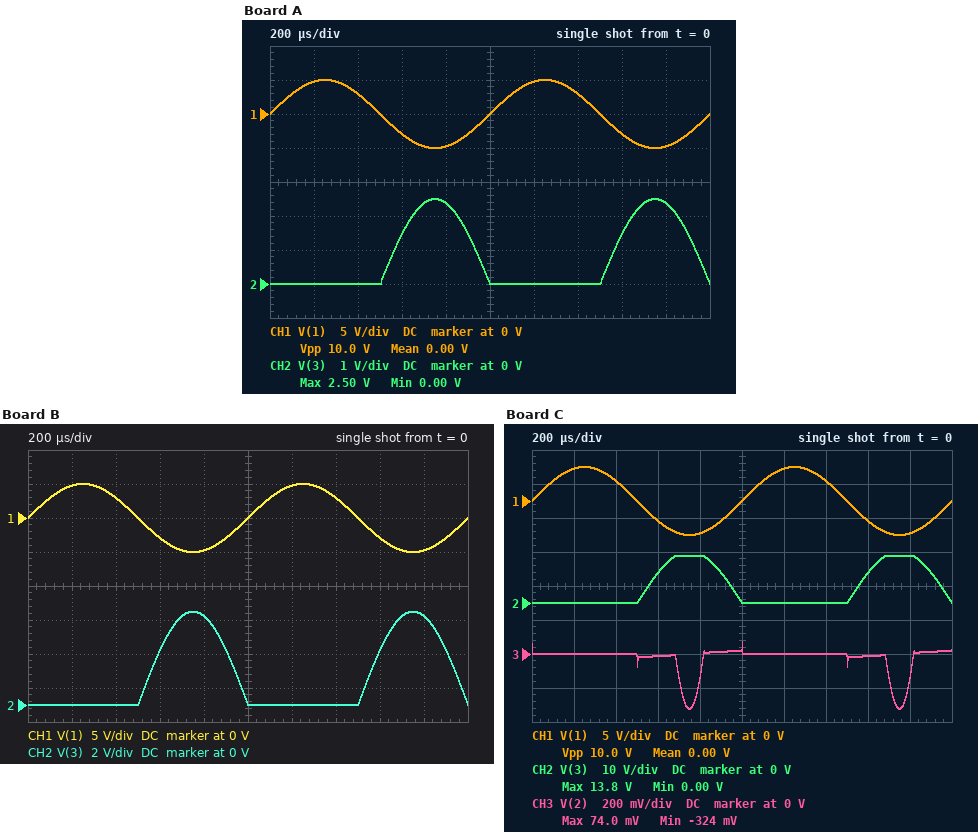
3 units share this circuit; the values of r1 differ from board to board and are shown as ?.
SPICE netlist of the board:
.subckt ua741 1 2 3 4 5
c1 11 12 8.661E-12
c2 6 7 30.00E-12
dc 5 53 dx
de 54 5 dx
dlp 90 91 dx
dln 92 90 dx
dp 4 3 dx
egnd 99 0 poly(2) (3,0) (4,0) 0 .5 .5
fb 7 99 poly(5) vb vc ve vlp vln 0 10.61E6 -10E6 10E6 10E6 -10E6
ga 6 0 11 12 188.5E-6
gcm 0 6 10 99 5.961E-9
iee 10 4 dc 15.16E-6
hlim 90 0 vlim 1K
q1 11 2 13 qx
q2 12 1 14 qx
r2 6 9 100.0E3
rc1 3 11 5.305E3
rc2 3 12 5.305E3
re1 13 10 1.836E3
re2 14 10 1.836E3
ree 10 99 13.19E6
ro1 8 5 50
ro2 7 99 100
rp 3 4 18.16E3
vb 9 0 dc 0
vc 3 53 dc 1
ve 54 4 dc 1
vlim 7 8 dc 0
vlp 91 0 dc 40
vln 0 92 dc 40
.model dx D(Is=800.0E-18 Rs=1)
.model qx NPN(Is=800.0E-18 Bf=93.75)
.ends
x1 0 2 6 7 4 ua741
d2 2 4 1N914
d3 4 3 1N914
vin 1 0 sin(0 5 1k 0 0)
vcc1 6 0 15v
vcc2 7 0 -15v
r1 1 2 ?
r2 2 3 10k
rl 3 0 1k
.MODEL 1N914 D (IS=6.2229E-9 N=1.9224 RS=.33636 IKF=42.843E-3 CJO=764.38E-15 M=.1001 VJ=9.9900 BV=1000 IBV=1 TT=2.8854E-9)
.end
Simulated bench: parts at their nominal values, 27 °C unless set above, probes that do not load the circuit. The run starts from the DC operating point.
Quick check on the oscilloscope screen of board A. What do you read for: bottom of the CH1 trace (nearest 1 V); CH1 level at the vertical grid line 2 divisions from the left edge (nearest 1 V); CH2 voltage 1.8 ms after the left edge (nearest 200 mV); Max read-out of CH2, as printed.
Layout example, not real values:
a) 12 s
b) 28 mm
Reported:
a) -5 V
b) 3 V
c) 2.4 V
d) 2.50 V
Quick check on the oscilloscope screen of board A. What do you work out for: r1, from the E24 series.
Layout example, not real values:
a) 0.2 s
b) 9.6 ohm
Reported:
a) 20 kΩ
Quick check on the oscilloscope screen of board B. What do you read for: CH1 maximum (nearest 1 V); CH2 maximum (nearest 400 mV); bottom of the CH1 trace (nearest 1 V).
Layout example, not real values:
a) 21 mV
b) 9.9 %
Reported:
a) 5 V
b) 5.6 V
c) -5 V
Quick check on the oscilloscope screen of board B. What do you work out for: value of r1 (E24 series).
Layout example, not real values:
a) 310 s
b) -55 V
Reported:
a) 9.1 kΩ
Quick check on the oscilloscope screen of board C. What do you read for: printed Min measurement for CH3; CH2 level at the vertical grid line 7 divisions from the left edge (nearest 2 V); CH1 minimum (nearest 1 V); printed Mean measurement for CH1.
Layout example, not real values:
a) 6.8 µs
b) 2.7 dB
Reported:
a) -324 mV
b) 0 V
c) -5 V
d) 0.00 V
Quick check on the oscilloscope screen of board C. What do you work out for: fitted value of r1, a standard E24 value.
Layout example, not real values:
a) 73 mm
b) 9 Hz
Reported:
a) 3.3 kΩ
